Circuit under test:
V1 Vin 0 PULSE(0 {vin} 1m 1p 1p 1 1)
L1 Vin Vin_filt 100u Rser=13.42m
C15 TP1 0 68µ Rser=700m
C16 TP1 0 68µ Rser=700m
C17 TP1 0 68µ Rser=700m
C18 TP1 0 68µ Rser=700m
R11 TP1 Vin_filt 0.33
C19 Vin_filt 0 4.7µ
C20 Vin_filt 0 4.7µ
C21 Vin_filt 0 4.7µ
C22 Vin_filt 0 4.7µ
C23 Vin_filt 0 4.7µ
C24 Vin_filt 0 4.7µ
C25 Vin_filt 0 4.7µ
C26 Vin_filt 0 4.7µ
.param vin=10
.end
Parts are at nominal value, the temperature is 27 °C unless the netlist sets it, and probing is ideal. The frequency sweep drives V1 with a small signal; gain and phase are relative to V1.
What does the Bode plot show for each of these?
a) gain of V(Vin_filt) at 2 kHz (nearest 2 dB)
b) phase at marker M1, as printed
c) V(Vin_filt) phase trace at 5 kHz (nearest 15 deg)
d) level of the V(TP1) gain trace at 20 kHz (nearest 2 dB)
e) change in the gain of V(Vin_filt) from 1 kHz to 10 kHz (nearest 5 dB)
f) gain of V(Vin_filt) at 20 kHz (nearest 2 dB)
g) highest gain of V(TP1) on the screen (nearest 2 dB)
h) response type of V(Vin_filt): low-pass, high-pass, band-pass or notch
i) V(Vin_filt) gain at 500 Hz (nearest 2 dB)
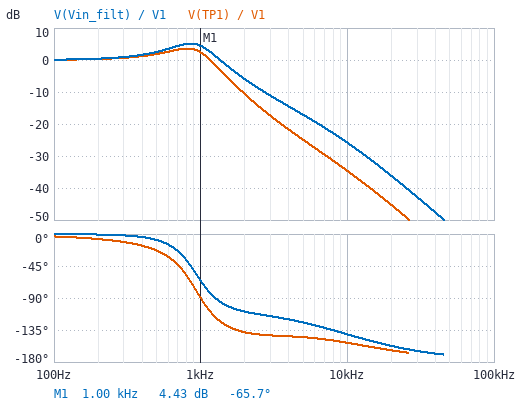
-6 dB
-65.7 deg
-120 deg
-46 dB
-30 dB
-36 dB
4 dB
low-pass
2 dB
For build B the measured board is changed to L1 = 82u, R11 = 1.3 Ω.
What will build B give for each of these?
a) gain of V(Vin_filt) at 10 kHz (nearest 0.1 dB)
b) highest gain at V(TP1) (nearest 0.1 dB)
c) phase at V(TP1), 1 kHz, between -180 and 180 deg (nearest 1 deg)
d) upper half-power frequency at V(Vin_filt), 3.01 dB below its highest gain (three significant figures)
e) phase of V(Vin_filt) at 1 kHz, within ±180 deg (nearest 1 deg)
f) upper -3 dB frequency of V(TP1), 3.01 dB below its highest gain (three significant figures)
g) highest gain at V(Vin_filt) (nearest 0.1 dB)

-21.5 dB
0 dB
-74 deg
3.06 kHz
-22 deg
490 Hz
2.2 dB
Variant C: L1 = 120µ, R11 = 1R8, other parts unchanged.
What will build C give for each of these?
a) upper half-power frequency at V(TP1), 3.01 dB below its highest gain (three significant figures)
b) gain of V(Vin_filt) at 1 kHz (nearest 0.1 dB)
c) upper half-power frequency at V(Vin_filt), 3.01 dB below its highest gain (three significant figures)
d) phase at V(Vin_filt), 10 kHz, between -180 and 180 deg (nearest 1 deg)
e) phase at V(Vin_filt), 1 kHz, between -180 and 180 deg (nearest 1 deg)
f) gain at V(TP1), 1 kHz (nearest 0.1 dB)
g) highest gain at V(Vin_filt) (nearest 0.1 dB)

349 Hz
1.9 dB
2.62 kHz
-167 deg
-26 deg
-8.7 dB
2.6 dB
